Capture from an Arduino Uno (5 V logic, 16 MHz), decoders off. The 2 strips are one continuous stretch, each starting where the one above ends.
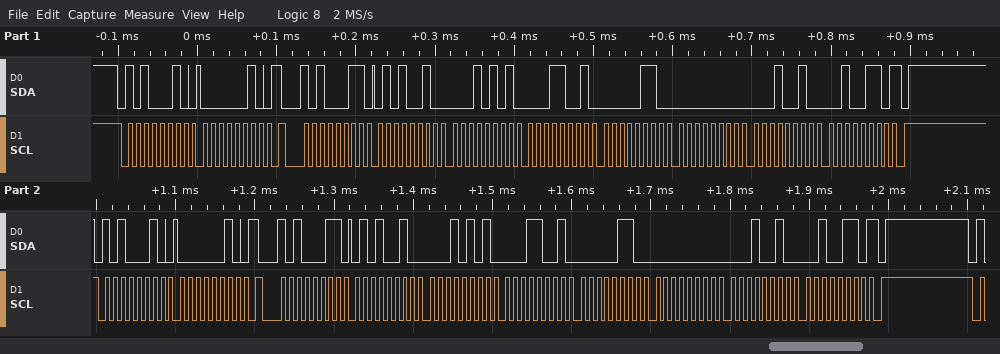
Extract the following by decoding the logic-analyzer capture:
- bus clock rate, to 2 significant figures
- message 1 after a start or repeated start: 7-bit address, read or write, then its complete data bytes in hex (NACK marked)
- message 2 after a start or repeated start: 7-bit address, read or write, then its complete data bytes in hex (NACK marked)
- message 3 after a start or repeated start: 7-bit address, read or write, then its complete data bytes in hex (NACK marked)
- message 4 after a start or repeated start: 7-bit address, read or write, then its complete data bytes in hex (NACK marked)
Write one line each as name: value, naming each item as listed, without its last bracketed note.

bus clock rate, to 2 significant figures: 100 kHz
message 1 after a start or repeated start: 7-bit address, read or write, then its complete data bytes in hex: 0x51 write: 02
message 2 after a start or repeated start: 7-bit address, read or write, then its complete data bytes in hex: 0x51 read: 52 15 19 06 00 12 26 NACK
message 3 after a start or repeated start: 7-bit address, read or write, then its complete data bytes in hex: 0x51 write: 02
message 4 after a start or repeated start: 7-bit address, read or write, then its complete data bytes in hex: 0x51 read: 52 15 19 06 00 12 26 NACK
